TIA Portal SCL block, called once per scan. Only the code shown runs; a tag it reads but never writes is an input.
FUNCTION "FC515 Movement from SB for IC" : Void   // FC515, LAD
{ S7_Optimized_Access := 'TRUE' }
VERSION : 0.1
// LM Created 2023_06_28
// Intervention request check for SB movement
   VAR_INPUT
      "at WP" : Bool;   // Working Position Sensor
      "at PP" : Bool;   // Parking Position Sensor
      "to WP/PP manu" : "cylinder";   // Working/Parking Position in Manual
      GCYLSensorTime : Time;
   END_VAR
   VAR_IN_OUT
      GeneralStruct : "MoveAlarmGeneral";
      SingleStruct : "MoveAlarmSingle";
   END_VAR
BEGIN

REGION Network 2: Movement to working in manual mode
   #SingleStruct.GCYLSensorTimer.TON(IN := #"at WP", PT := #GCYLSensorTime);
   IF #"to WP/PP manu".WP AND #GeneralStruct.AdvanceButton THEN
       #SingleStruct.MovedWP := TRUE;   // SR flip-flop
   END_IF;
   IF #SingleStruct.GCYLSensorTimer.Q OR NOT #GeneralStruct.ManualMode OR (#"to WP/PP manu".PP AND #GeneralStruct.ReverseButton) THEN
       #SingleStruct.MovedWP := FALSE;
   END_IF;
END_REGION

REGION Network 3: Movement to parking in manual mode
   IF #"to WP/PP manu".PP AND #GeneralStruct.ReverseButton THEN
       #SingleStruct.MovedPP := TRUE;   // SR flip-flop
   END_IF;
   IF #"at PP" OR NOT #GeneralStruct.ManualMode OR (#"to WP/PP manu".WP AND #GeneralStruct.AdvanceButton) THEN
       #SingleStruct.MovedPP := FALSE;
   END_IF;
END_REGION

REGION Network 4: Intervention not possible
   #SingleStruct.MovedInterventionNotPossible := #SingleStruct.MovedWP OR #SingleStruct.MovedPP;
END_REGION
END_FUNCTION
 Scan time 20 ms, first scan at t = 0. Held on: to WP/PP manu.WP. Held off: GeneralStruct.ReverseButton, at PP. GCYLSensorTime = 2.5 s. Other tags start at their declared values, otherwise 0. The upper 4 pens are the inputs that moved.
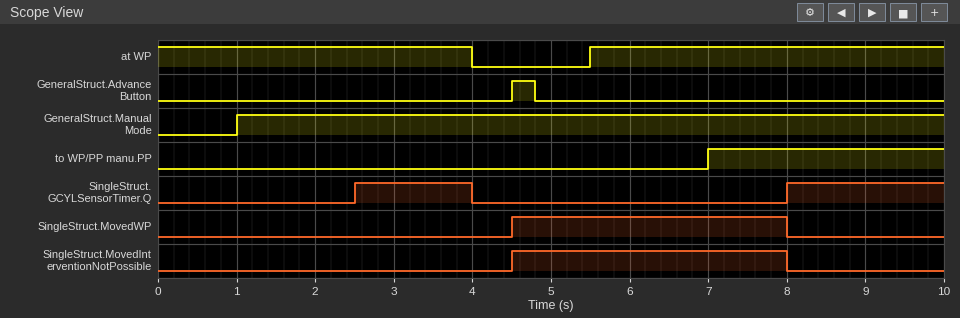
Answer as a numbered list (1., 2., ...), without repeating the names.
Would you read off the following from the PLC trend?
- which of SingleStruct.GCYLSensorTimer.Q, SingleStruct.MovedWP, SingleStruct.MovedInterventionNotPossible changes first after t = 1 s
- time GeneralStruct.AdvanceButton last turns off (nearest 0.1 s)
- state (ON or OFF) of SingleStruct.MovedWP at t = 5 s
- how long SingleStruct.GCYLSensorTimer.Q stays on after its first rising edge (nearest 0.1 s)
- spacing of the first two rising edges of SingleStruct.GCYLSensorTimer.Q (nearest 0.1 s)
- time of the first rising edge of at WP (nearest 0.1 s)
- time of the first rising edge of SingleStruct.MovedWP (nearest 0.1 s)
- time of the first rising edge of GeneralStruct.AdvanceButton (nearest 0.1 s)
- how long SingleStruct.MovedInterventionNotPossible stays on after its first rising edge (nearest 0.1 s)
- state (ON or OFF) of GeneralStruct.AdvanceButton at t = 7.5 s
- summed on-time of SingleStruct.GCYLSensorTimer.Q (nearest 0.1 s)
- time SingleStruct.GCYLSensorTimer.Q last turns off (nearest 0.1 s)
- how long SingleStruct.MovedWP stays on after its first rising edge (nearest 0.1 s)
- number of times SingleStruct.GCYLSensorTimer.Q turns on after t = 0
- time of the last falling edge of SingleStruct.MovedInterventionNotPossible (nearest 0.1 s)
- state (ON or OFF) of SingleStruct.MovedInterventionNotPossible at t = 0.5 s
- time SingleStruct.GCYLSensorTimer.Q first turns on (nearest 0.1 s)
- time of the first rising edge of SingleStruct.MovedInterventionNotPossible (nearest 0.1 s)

1. SingleStruct.GCYLSensorTimer.Q
2. 4.8 s
3. ON
4. 1.5 s
5. 5.5 s
6. 5.5 s
7. 4.5 s
8. 4.5 s
9. 3.5 s
10. OFF
11. 3.5 s
12. 4.0 s
13. 3.5 s
14. 2
15. 8.0 s
16. OFF
17. 2.5 s
18. 4.5 s
